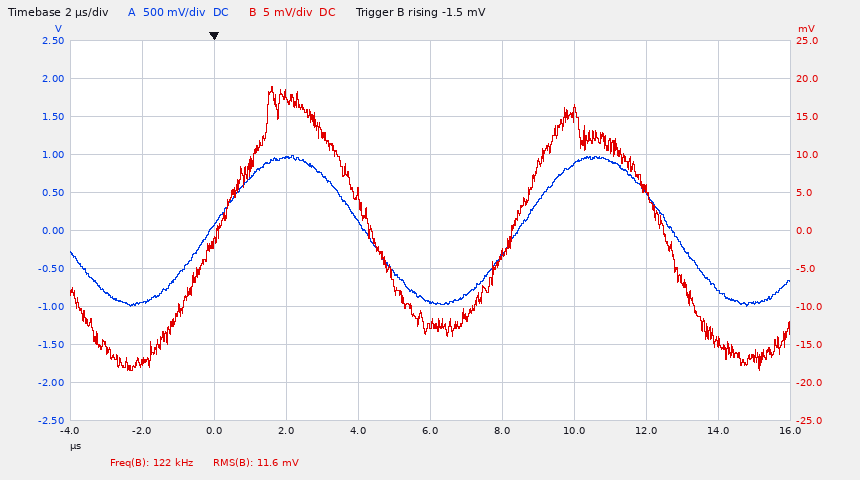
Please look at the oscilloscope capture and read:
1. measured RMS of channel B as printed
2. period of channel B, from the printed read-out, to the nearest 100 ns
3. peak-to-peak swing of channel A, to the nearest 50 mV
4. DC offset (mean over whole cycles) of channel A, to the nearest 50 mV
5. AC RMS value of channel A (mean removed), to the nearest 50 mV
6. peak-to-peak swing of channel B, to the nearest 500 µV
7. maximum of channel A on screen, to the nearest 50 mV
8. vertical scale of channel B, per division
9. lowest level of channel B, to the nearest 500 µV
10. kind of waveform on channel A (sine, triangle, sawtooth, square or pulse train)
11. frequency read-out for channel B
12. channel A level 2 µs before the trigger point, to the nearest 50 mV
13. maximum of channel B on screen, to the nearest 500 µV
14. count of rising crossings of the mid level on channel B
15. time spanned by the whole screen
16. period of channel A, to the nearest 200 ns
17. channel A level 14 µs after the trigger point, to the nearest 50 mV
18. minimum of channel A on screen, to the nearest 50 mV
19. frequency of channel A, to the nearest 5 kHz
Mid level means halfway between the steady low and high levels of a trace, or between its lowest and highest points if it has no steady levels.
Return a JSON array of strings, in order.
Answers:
["11.6 mV", "8.2 µs", "2.00 V", "0 mV", "700 mV", "37.5 mV", "1.00 V", "5 mV", "-18.5 mV", "sine", "122 kHz", "-950 mV", "19.0 mV", "2", "20 µs", "8.6 µs", "-800 mV", "-1.00 V", "115 kHz"]
